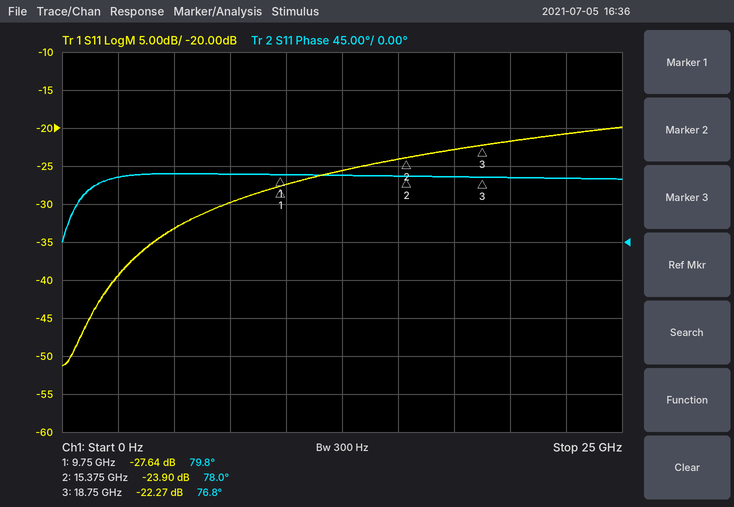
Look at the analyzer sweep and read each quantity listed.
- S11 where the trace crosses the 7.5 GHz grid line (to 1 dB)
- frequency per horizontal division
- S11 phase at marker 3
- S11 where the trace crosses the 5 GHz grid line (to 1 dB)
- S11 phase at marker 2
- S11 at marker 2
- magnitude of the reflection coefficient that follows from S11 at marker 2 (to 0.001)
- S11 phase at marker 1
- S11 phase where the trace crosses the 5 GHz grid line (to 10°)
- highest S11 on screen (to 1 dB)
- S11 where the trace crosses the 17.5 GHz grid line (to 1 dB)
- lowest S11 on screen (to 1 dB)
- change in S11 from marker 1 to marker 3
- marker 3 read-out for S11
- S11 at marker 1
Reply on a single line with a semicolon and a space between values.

-30 dB; 2.5 GHz; 76.8°; -33 dB; 78.0°; -23.90 dB; 0.064; 79.8°; 80°; -20 dB; -23 dB; -51 dB; 5.37 dB; -22.27 dB; -27.64 dB
